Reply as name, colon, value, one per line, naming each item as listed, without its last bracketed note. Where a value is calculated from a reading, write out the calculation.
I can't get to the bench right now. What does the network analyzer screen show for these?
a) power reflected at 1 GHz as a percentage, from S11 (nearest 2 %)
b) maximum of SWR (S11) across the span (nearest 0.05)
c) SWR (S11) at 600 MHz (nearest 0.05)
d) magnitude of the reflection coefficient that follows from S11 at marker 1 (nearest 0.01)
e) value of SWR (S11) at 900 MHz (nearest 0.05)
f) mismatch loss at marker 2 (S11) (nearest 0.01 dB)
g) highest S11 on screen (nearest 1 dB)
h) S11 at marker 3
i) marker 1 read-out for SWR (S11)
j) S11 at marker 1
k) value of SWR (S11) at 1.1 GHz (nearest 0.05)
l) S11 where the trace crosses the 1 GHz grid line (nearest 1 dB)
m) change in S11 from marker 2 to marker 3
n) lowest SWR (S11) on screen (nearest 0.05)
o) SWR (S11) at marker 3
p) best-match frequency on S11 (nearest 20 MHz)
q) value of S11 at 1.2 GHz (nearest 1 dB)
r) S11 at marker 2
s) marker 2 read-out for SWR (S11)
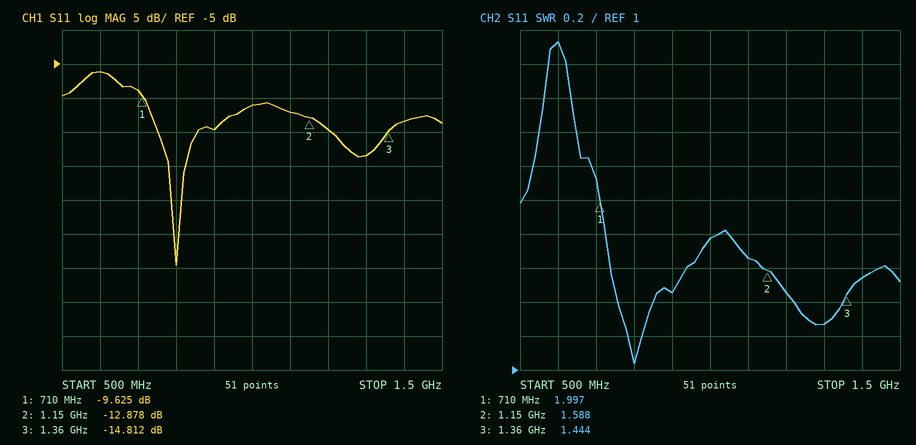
power reflected at 1 GHz as a percentage, from S11: 10^(-11/10) ≈ 8 %
maximum of SWR (S11) across the span: 2.95
SWR (S11) at 600 MHz: 2.95
magnitude of the reflection coefficient that follows from S11 at marker 1: 10^(-9.625/20) ≈ 0.33
value of SWR (S11) at 900 MHz: 1.45
mismatch loss at marker 2 (S11): −10 log10(1 − 10^(-12.878/10)) ≈ 0.23 dB
highest S11 on screen: -6 dB
S11 at marker 3: -14.812 dB
marker 1 read-out for SWR: 1.997
S11 at marker 1: -9.625 dB
value of SWR (S11) at 1.1 GHz: 1.65
S11 where the trace crosses the 1 GHz grid line: -11 dB
change in S11 from marker 2 to marker 3: -14.812 − (-12.878) = -1.934 dB
lowest SWR (S11) on screen: 1.05
SWR (S11) at marker 3: 1.444
best-match frequency on S11: 800 MHz
value of S11 at 1.2 GHz: -15 dB
S11 at marker 2: -12.878 dB
marker 2 read-out for SWR: 1.588
